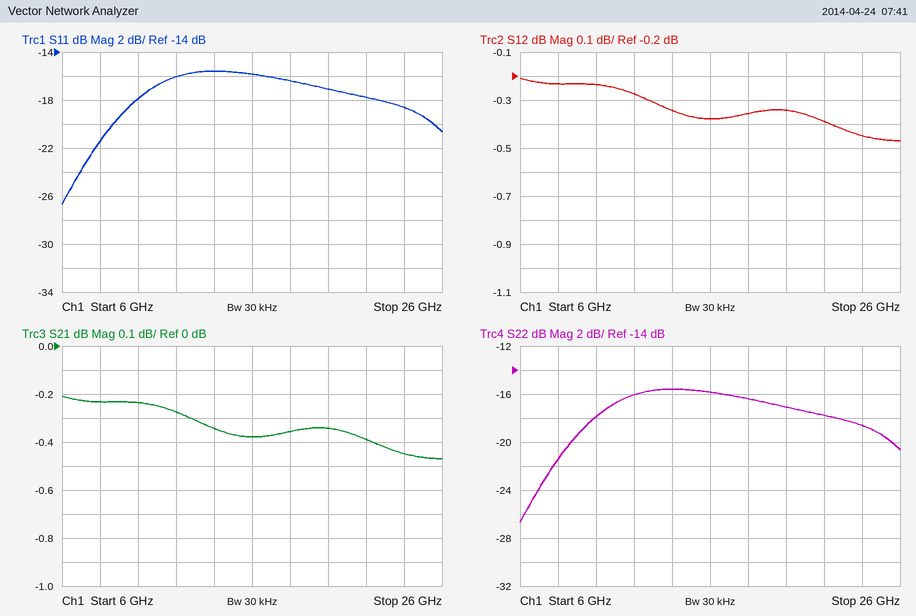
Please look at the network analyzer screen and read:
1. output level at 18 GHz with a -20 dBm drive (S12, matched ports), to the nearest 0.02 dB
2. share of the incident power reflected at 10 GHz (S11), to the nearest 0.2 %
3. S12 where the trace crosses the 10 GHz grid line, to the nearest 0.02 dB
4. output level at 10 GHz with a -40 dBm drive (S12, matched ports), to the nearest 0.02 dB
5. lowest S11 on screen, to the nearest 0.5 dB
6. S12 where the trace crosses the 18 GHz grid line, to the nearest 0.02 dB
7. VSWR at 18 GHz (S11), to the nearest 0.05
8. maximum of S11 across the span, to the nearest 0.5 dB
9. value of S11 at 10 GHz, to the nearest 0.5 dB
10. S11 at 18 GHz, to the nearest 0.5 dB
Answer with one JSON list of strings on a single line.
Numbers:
["-20.36 dBm", "1.6 %", "-0.24 dB", "-40.24 dBm", "-26.5 dB", "-0.36 dB", "1.35", "-15.5 dB", "-18.0 dB", "-16.5 dB"]
